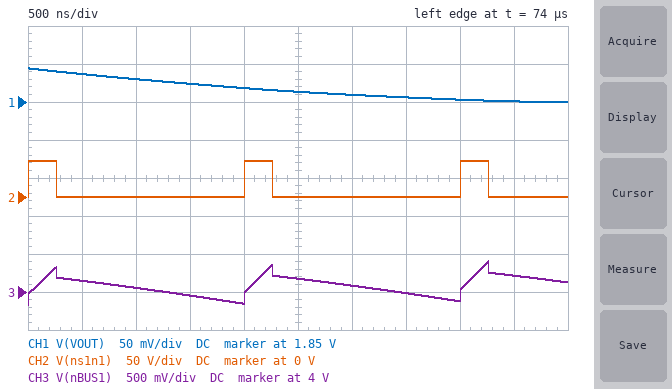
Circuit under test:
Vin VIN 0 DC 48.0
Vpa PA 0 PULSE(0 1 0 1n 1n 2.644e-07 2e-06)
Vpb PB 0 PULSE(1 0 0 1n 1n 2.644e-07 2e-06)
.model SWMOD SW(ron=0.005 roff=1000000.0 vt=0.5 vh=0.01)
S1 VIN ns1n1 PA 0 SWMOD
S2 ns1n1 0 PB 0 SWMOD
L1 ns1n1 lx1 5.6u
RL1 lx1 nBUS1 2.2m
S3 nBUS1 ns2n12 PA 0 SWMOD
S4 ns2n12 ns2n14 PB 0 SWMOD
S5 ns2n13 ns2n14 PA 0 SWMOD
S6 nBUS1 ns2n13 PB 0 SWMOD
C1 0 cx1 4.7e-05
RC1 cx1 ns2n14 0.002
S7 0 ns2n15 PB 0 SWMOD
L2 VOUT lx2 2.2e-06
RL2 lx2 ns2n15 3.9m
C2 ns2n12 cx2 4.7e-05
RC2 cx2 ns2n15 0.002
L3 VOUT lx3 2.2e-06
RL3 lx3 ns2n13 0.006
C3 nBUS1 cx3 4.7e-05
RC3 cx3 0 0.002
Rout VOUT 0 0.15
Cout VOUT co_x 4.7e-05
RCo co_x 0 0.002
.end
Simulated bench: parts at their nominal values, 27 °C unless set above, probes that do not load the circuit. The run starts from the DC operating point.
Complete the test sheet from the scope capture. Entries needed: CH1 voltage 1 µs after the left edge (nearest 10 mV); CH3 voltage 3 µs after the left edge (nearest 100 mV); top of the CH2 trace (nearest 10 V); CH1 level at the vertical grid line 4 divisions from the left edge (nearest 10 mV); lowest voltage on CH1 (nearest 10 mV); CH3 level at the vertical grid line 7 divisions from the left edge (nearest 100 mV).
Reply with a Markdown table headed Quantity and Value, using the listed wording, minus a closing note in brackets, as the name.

| Quantity | Value |
|---|---|
| CH1 voltage 1 µs after the left edge | 1.88 V |
| CH3 voltage 3 µs after the left edge | 4.1 V |
| top of the CH2 trace | 50 V |
| CH1 level at the vertical grid line 4 divisions from the left edge | 1.87 V |
| lowest voltage on CH1 | 1.85 V |
| CH3 level at the vertical grid line 7 divisions from the left edge | 4.0 V |
